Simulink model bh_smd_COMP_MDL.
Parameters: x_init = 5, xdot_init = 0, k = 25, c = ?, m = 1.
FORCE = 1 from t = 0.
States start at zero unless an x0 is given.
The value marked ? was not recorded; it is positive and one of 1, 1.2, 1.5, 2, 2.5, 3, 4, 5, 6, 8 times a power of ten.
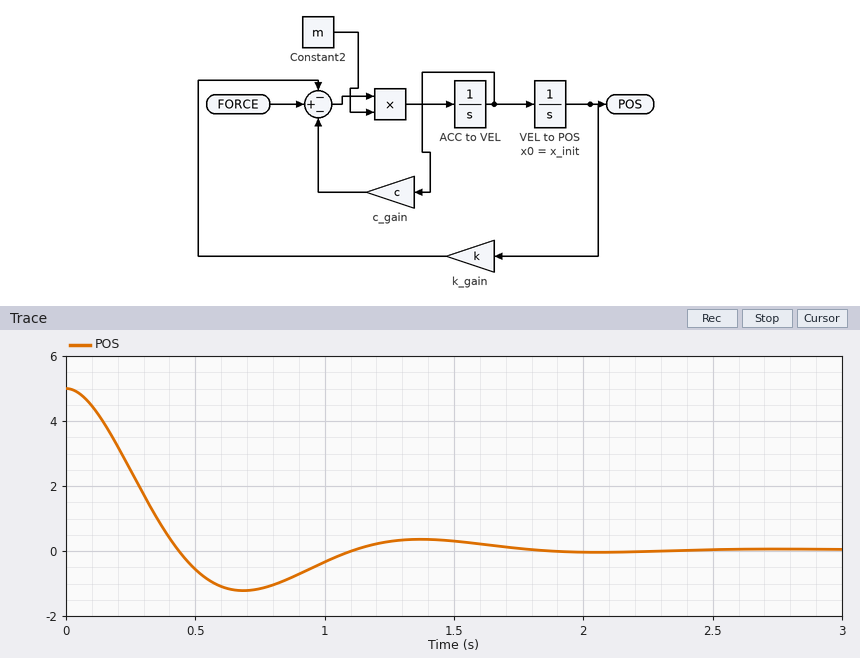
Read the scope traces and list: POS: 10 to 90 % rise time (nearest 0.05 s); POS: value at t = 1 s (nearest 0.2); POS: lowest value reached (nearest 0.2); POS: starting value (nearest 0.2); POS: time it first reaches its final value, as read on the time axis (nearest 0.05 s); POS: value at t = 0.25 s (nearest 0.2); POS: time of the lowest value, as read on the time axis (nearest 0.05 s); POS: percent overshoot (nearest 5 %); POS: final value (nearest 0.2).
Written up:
0.30 s
-0.4
-1.2
5.0
0.45 s
2.4
0.70 s
25 %
0.0
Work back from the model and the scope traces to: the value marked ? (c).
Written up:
4
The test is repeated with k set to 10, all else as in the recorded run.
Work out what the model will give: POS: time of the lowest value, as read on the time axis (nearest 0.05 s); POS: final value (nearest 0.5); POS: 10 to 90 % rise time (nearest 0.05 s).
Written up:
1.30 s
0.0
0.60 s
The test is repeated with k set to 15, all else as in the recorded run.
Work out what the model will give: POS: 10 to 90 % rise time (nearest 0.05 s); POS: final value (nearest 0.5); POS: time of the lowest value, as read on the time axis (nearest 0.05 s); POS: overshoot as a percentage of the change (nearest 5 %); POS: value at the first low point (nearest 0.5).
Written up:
0.45 s
0.0
0.95 s
15 %
-0.5
